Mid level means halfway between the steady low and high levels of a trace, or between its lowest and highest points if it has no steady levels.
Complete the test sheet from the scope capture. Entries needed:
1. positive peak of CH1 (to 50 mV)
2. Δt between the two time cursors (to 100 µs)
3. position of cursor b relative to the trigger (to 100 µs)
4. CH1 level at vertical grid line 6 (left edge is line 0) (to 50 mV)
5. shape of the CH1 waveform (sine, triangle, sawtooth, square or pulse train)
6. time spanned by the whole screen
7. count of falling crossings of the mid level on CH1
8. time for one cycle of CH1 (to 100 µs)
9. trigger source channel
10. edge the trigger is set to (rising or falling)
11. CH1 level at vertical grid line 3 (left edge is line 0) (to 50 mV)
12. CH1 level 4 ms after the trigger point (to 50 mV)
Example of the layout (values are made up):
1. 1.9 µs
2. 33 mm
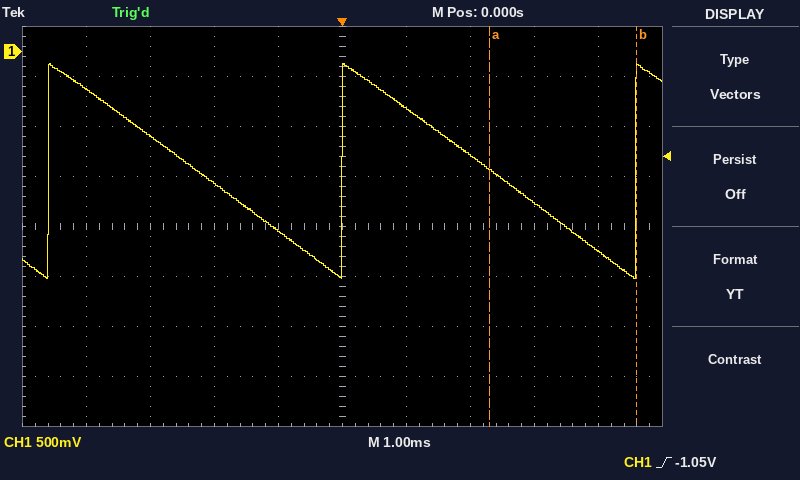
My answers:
1. -100 mV
2. 2.3 ms
3. +4.6 ms
4. -550 mV
5. sawtooth
6. 10 ms
7. 2
8. 4.6 ms
9. CH1
10. rising
11. -1.30 V
12. -2.00 V
